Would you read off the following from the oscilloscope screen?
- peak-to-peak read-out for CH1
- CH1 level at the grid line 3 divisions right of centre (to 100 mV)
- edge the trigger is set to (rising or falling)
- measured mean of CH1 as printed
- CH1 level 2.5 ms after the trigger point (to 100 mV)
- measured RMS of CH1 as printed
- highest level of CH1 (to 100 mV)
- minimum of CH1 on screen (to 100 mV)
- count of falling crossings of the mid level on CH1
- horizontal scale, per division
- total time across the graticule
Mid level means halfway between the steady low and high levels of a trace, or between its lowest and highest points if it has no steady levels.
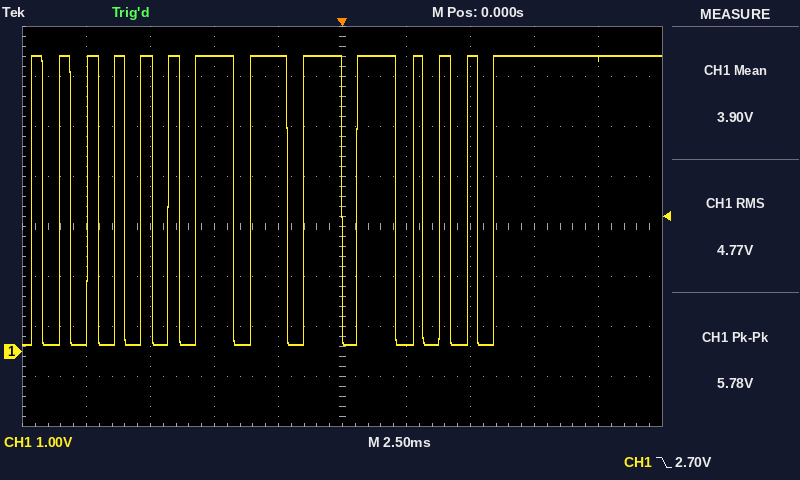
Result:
5.78 V
5.9 V
falling
3.90 V
100 mV
4.77 V
5.9 V
100 mV
13
2.5 ms
25 ms
